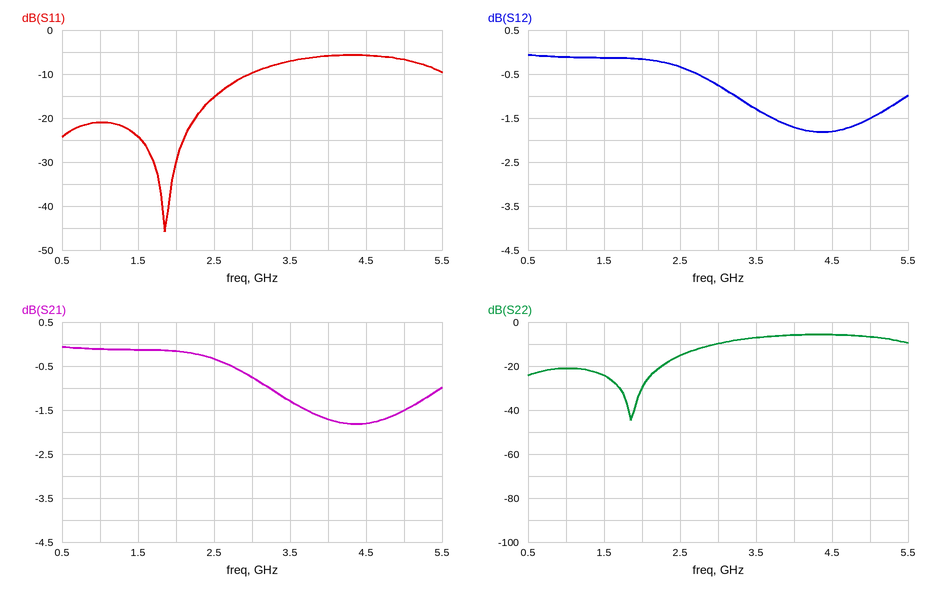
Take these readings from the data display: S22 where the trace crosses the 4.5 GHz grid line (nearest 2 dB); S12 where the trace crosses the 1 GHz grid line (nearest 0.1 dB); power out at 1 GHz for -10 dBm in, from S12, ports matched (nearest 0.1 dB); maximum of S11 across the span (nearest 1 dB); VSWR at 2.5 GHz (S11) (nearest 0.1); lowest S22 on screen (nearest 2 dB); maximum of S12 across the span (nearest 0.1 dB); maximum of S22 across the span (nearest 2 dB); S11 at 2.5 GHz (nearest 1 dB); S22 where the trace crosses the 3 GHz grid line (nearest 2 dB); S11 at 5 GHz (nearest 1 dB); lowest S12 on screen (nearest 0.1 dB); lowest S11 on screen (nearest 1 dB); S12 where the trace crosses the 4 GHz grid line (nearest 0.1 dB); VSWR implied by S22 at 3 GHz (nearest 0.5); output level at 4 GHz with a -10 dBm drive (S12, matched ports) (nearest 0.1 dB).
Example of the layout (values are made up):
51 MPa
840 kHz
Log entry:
-6 dB
-0.1 dB
-10.1 dBm
-6 dB
1.4
-44 dB
-0.1 dB
-6 dB
-15 dB
-10 dB
-7 dB
-1.8 dB
-46 dB
-1.7 dB
2.0
-11.7 dBm
